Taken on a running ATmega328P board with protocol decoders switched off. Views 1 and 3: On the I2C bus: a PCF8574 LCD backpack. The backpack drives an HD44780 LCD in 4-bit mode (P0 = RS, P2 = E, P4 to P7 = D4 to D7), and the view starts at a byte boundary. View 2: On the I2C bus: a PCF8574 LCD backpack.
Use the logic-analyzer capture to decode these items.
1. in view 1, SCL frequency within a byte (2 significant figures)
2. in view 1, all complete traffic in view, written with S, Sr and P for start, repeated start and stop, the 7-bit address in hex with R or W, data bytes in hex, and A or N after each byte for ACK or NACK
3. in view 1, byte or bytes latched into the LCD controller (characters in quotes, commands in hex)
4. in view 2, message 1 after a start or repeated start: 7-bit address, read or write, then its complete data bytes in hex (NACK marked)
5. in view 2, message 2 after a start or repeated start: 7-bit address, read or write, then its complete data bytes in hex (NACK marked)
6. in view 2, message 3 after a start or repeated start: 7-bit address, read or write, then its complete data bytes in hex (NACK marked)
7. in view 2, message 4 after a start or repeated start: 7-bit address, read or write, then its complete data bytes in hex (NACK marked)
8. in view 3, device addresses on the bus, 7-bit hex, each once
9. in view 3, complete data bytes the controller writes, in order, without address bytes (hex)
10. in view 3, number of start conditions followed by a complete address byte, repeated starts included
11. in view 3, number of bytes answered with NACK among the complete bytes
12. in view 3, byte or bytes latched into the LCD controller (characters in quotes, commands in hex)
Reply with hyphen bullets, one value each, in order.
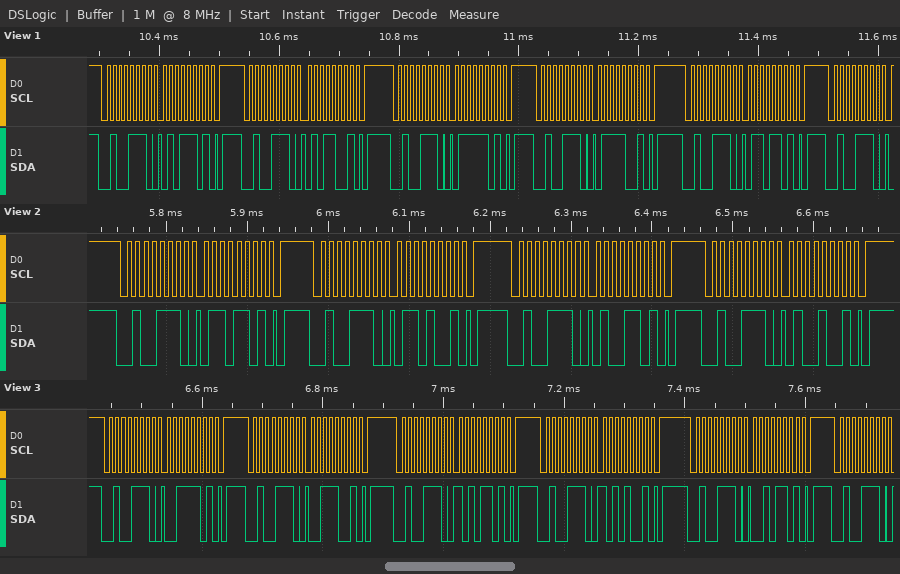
- 100 kHz
- S 27W A 5D A P S 27W A 59 A P S 27W A 7D A P S 27W A 79 A P S 27W A 6D A P S 27W A
- 'W'
- 0x27 write: 6D
- 0x27 write: 69
- 0x27 write: 4D
- 0x27 write: 49
- 0x27
- 3D 39 AD A9 2D
- 6
- 0
- ':'
